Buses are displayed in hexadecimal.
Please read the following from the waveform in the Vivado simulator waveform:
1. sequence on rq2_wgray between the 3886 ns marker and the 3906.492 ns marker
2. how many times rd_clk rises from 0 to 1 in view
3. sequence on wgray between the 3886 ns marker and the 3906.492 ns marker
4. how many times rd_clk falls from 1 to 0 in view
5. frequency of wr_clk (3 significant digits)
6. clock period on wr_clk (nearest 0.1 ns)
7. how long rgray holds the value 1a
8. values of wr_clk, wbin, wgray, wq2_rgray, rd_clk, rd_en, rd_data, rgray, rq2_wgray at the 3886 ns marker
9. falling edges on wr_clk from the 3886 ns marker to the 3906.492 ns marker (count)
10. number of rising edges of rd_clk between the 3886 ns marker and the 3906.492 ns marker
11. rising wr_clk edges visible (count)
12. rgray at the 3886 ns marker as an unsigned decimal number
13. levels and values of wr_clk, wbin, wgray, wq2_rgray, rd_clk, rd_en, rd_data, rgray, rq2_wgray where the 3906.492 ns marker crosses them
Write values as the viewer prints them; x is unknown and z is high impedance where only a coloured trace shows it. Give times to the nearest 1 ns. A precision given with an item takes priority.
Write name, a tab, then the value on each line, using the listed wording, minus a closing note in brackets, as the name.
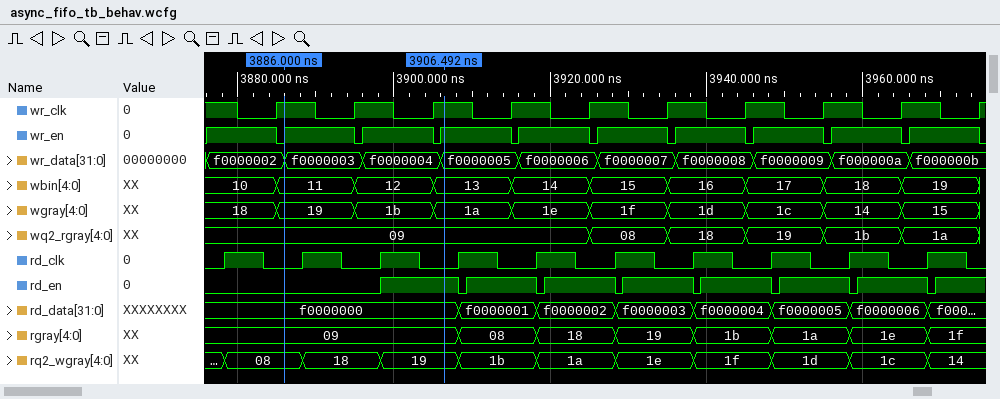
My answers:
sequence on rq2_wgray between the 3886 ns marker and the 3906.492 ns marker	08, 18, 19
how many times rd_clk rises from 0 to 1 in view	10
sequence on wgray between the 3886 ns marker and the 3906.492 ns marker	19, 1b, 1a
how many times rd_clk falls from 1 to 0 in view	10
frequency of wr_clk	100 MHz
clock period on wr_clk	10 ns
how long rgray holds the value 1a	10 ns
values of wr_clk, wbin, wgray, wq2_rgray, rd_clk, rd_en, rd_data, rgray, rq2_wgray at the 3886 ns marker	wr_clk=1, wbin=11, wgray=19, wq2_rgray=09, rd_clk=0, rd_en=0, rd_data=f0000000, rgray=09, rq2_wgray=08
falling edges on wr_clk from the 3886 ns marker to the 3906.492 ns marker	2
number of rising edges of rd_clk between the 3886 ns marker and the 3906.492 ns marker	2
rising wr_clk edges visible	10
rgray at the 3886 ns marker as an unsigned decimal number	9
levels and values of wr_clk, wbin, wgray, wq2_rgray, rd_clk, rd_en, rd_data, rgray, rq2_wgray where the 3906.492 ns marker crosses them	wr_clk=1, wbin=13, wgray=1a, wq2_rgray=09, rd_clk=0, rd_en=1, rd_data=f0000000, rgray=09, rq2_wgray=19
